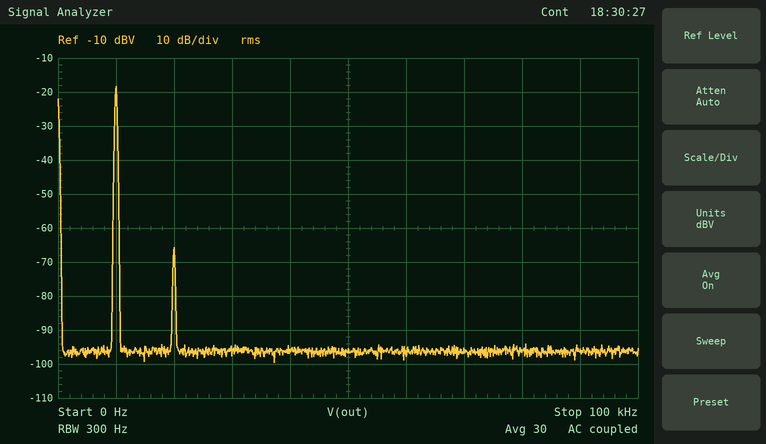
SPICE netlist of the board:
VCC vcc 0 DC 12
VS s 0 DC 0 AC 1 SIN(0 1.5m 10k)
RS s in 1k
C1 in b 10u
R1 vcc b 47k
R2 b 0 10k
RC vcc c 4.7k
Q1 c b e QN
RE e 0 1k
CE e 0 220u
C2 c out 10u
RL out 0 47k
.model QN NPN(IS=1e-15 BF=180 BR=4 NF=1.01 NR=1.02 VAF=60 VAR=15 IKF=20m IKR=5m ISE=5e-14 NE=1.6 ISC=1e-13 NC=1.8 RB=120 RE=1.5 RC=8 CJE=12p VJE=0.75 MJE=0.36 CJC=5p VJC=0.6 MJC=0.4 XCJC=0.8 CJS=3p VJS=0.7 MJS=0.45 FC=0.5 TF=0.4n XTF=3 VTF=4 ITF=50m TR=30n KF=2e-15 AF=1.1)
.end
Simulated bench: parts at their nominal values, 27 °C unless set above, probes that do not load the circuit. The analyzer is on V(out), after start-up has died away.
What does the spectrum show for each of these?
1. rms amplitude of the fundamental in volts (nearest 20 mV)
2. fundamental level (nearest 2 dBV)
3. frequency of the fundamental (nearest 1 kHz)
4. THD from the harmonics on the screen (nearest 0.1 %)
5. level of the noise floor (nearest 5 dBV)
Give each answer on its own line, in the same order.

120 mV
-18 dBV
10 kHz
0.4 %
-95 dBV
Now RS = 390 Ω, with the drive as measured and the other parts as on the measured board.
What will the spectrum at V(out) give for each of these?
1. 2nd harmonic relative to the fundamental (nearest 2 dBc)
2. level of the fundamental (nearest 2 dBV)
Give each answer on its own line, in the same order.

-44 dBc
-16 dBV
